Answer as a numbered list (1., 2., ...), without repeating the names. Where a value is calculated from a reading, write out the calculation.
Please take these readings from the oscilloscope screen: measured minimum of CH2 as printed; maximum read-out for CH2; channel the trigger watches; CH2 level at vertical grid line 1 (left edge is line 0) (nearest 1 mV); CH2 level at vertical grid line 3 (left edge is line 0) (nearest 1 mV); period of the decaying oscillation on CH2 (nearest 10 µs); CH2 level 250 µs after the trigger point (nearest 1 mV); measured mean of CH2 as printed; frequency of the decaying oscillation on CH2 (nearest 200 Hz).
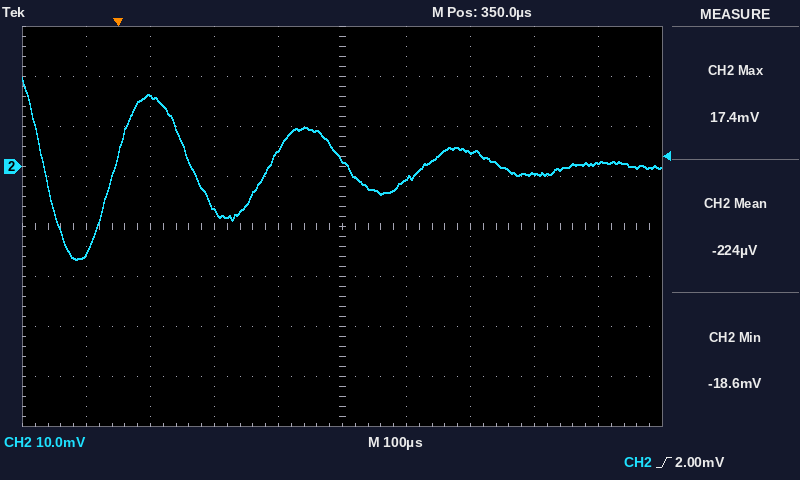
1. -18.6 mV
2. 17.4 mV
3. CH2
4. -17 mV
5. -9 mV
6. 240 µs
7. 3 mV
8. -224 µV
9. 1 / 240 µs ≈ 4.2 kHz
